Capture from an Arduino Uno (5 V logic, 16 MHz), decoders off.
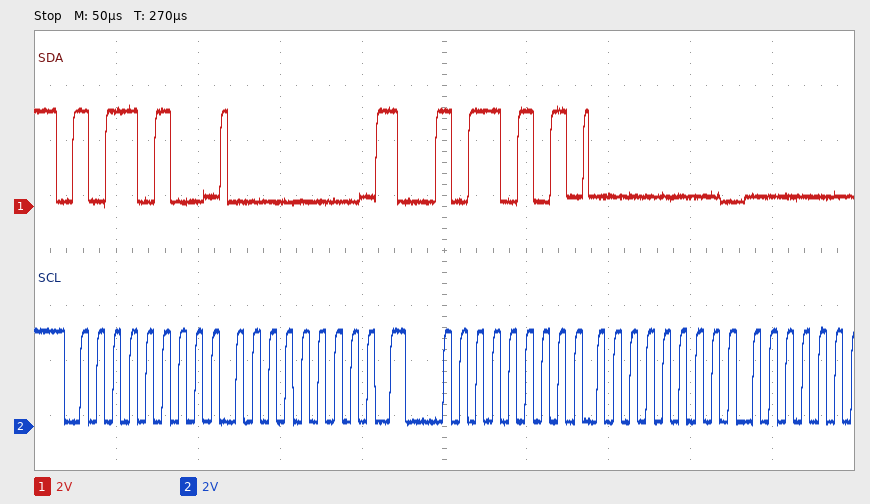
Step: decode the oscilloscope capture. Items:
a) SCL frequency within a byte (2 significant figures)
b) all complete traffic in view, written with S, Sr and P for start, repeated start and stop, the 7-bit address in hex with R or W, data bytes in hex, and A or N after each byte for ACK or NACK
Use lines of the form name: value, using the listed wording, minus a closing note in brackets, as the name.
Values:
SCL frequency within a byte: 100 kHz
all complete traffic in view, written with S, Sr and P for start, repeated start and stop, the 7-bit address in hex with R or W, data bytes in hex, and A or N after each byte for ACK or NACK: S 5AW A 00 A Sr 5AR A 00 A
